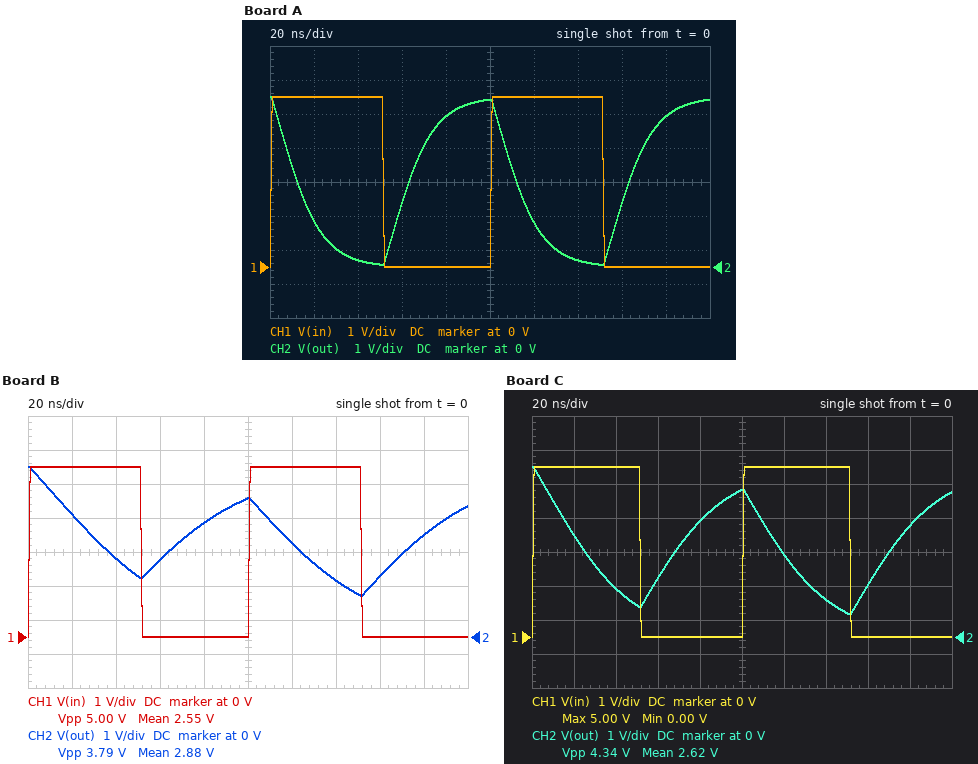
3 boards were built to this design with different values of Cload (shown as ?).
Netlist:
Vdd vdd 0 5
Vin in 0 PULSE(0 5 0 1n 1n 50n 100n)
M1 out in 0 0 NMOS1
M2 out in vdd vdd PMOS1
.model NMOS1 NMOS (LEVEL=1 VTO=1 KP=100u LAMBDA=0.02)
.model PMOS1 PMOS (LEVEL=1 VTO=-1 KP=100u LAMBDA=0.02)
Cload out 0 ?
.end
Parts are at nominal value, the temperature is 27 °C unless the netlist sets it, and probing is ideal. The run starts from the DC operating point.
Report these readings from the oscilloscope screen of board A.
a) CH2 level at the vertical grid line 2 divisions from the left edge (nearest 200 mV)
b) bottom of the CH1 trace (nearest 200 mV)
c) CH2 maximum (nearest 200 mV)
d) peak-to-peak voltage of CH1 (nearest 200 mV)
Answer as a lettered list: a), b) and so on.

a) 200 mV
b) 0 V
c) 5.0 V
d) 5.0 V
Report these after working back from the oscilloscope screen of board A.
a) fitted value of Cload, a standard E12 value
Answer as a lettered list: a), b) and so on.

a) 3.9 pF
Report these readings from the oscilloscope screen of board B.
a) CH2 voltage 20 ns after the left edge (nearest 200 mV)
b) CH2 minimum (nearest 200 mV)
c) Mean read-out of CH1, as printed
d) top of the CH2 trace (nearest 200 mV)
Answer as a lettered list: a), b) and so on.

a) 3.6 V
b) 1.2 V
c) 2.55 V
d) 5.0 V
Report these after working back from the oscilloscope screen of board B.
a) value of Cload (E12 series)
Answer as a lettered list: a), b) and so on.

a) 12 pF
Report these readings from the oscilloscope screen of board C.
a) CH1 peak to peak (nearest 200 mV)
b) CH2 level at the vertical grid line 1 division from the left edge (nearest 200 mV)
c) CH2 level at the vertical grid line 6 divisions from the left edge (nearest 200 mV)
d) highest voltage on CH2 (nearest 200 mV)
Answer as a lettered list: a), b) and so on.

a) 5.0 V
b) 3.0 V
c) 2.4 V
d) 5.0 V
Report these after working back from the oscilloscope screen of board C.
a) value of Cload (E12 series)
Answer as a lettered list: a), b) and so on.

a) 8.2 pF
